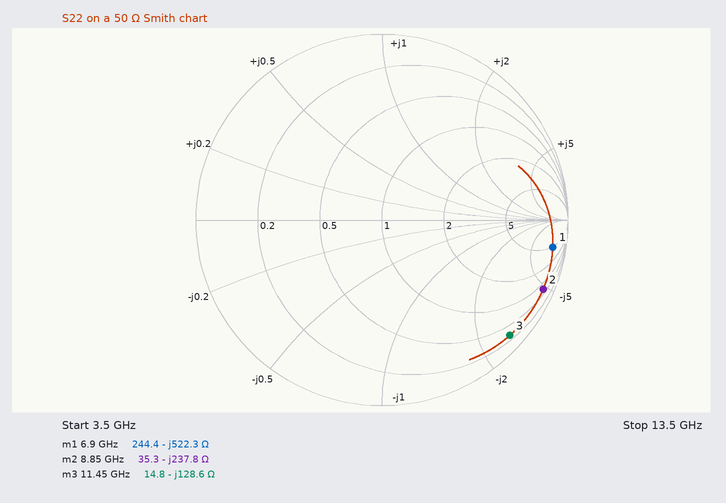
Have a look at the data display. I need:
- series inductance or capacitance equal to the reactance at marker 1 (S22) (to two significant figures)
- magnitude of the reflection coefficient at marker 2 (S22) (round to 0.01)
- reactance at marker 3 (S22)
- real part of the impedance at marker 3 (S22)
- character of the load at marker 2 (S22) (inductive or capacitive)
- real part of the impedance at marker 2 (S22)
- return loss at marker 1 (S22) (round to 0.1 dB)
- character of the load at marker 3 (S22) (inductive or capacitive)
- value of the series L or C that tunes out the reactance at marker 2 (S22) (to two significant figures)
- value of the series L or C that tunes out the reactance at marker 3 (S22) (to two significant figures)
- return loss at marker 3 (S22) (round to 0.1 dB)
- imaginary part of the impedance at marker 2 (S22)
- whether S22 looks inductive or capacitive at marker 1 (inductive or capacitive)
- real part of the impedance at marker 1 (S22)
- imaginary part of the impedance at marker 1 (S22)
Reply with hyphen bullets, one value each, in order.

- 44 fF
- 0.94
- -128.6 Ω
- 14.8 Ω
- capacitive
- 35.3 Ω
- 0.6 dB
- capacitive
- 4.3 nH
- 1.8 nH
- 0.7 dB
- -237.8 Ω
- capacitive
- 244.4 Ω
- -522.3 Ω
